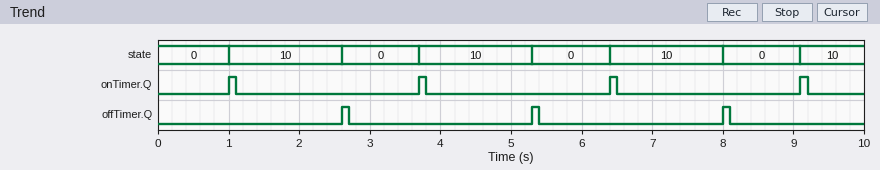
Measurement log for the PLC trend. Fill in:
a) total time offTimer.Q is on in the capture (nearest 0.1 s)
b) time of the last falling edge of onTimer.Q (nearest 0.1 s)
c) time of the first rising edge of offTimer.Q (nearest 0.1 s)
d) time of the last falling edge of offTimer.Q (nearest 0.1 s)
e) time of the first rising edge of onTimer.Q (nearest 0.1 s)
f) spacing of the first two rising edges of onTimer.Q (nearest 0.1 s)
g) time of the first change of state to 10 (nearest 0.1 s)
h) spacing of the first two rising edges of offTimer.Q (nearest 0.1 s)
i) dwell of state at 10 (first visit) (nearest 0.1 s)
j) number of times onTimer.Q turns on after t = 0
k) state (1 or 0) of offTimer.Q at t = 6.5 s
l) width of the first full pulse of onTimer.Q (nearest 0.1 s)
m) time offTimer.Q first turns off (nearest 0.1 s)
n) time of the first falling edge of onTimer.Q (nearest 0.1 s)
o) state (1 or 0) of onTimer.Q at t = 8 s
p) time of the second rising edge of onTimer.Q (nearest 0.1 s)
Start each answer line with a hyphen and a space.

- 0.3 s
- 9.2 s
- 2.6 s
- 8.1 s
- 1.0 s
- 2.7 s
- 1.0 s
- 2.7 s
- 1.6 s
- 4
- 0
- 0.1 s
- 2.7 s
- 1.1 s
- 0
- 3.7 s
